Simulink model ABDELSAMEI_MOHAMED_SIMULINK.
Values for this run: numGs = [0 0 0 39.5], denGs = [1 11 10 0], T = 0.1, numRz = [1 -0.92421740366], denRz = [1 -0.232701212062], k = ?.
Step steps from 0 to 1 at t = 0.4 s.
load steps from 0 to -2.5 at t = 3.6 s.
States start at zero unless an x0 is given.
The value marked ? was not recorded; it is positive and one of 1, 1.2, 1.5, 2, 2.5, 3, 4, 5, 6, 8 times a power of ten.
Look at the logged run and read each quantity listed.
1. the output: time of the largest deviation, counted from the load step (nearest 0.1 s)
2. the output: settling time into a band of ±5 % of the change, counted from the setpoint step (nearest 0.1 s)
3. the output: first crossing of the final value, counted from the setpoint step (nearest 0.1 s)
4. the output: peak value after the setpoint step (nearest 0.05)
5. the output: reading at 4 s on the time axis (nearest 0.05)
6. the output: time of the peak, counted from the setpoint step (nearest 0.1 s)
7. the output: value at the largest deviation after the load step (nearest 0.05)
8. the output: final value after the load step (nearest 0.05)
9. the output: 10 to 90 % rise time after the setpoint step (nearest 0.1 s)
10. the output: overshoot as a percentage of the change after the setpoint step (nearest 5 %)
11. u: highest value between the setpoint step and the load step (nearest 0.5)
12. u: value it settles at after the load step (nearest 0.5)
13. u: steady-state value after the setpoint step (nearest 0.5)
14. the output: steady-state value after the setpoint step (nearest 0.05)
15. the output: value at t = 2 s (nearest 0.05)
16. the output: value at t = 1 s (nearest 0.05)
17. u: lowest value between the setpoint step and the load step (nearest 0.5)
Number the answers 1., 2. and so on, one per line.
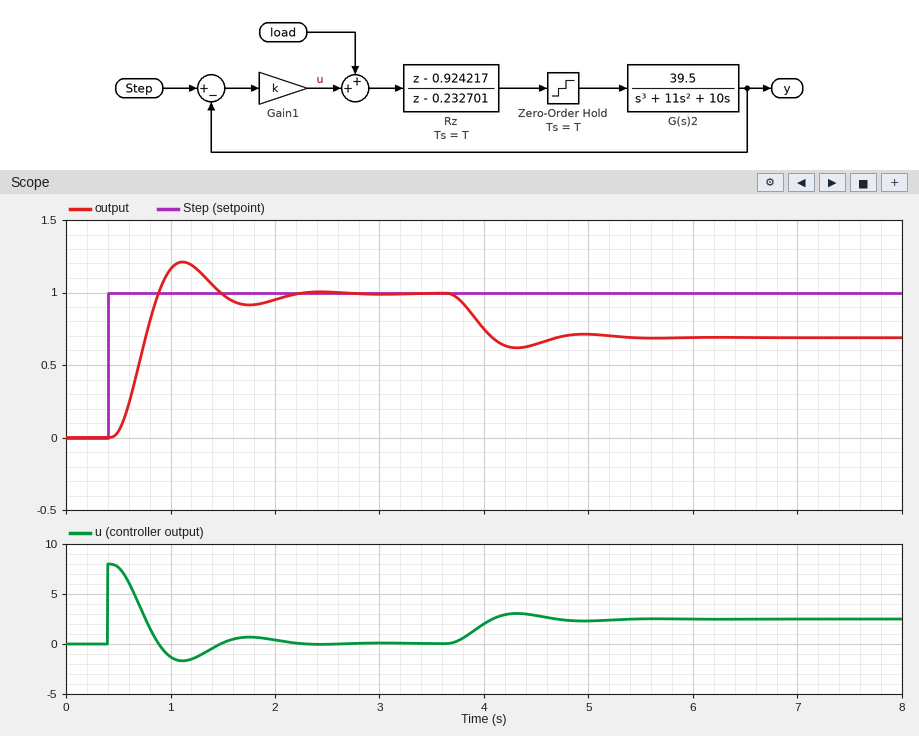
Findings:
1. 0.7 s
2. 1.6 s
3. 0.5 s
4. 1.20
5. 0.75
6. 0.7 s
7. 0.60
8. 0.70
9. 0.3 s
10. 20 %
11. 8.0
12. 2.5
13. 0.0
14. 1.00
15. 0.95
16. 1.15
17. -1.5
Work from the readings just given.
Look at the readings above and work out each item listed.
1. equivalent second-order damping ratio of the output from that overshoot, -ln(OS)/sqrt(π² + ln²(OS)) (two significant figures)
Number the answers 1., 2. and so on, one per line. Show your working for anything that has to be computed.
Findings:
1. ln(0.2) = -1.609; 1.609 / sqrt(9.870 + 2.590) = 0.46
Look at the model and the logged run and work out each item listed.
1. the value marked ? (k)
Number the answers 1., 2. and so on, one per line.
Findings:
1. 8
